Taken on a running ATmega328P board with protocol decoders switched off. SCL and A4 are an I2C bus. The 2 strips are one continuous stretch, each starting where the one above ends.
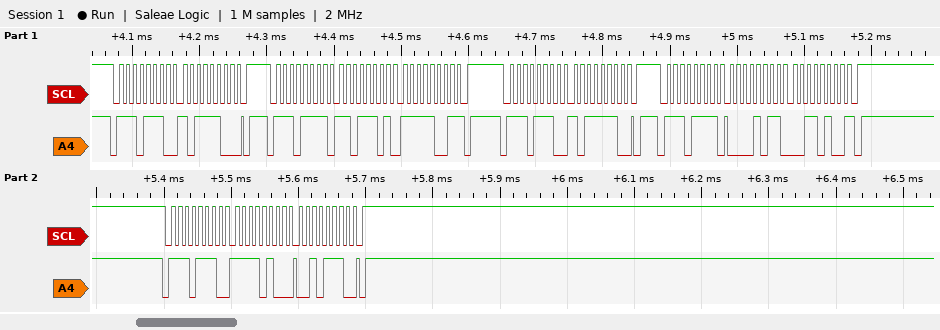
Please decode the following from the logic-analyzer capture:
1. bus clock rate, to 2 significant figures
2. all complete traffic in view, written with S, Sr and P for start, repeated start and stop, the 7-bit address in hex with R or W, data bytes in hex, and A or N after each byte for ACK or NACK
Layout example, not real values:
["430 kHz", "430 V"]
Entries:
["100 kHz", "S 77W A BC A P S 77R A DD A F9 N P S 77W A BE A P S 77R A 0B A 34 N P S 77W A F4 A 2E A P"]
